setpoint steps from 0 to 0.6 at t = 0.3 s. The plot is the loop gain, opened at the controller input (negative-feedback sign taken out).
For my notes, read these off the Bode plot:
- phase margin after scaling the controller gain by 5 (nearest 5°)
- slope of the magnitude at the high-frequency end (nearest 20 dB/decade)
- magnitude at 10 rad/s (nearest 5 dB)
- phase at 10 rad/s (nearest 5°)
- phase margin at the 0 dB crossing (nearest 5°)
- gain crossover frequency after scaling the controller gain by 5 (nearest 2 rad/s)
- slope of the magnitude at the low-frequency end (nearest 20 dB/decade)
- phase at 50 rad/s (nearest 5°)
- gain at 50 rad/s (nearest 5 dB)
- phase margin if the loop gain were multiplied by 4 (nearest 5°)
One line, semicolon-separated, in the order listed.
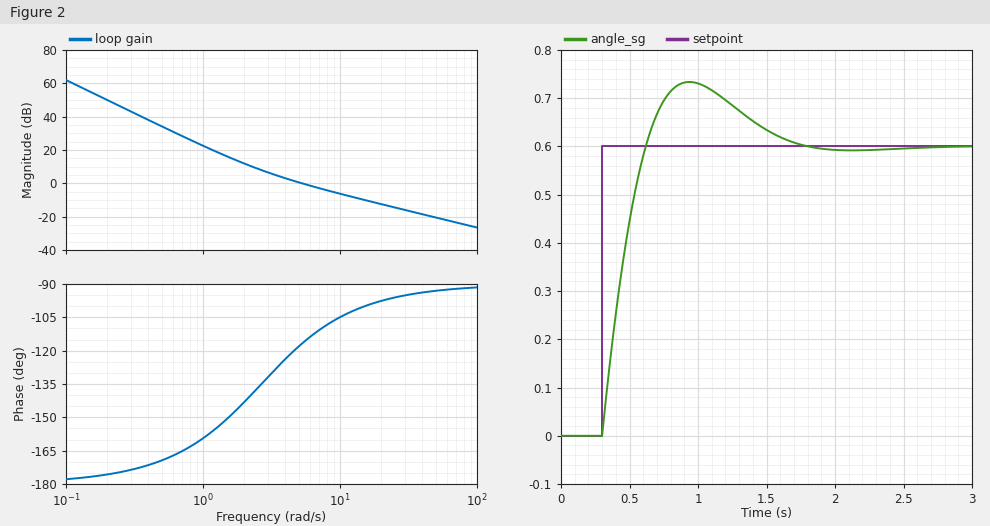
85°; -20 dB/decade; -5 dB; -105°; 65°; 24 rad/s; -40 dB/decade; -95°; -20 dB; 80°
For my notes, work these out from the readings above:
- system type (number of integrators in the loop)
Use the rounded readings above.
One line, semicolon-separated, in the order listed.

2
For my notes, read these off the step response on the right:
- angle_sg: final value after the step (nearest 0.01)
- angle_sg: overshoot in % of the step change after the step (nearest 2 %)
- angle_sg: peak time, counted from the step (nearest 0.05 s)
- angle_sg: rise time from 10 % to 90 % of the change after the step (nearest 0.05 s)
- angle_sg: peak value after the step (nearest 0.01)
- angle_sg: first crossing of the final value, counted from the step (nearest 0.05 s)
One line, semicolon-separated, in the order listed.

0.60; 22 %; 0.65 s; 0.25 s; 0.73; 0.30 s
